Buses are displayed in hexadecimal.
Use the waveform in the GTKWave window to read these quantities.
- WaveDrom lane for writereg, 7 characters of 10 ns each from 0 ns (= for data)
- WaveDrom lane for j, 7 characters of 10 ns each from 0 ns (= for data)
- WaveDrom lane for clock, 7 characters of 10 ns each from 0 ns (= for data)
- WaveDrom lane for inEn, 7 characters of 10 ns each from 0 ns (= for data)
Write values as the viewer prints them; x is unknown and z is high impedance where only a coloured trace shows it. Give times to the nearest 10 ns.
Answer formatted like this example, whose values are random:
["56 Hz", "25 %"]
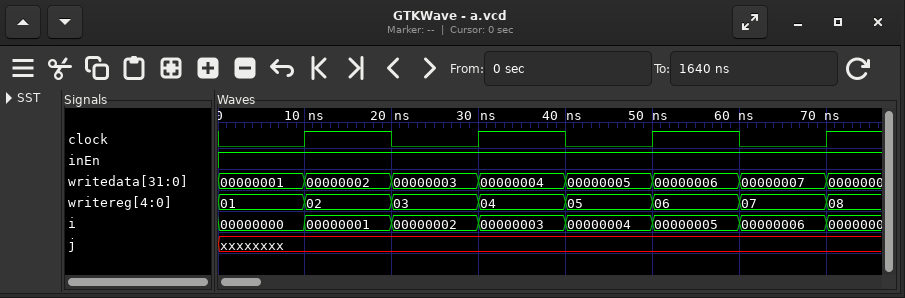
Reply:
["{name: 'writereg', wave: '=======', data: '01 02 03 04 05 06 07'}", "{name: 'j', wave: 'x......'}", "{name: 'clock', wave: '0101010'}", "{name: 'inEn', wave: '1......'}"]
